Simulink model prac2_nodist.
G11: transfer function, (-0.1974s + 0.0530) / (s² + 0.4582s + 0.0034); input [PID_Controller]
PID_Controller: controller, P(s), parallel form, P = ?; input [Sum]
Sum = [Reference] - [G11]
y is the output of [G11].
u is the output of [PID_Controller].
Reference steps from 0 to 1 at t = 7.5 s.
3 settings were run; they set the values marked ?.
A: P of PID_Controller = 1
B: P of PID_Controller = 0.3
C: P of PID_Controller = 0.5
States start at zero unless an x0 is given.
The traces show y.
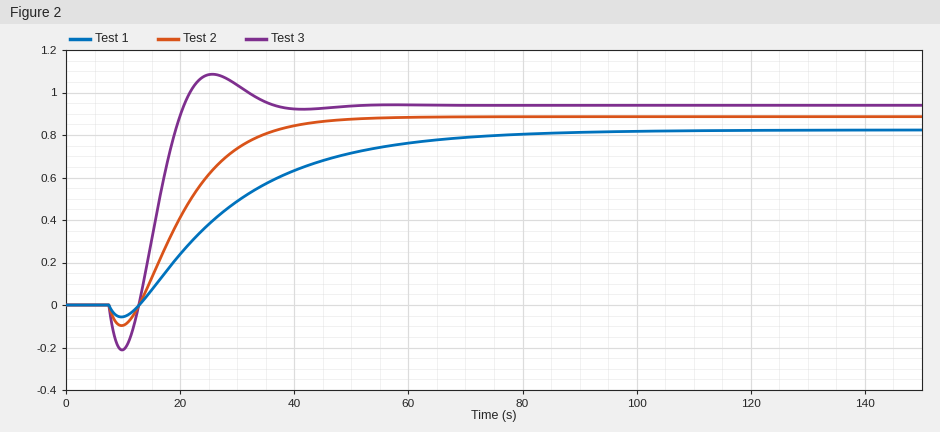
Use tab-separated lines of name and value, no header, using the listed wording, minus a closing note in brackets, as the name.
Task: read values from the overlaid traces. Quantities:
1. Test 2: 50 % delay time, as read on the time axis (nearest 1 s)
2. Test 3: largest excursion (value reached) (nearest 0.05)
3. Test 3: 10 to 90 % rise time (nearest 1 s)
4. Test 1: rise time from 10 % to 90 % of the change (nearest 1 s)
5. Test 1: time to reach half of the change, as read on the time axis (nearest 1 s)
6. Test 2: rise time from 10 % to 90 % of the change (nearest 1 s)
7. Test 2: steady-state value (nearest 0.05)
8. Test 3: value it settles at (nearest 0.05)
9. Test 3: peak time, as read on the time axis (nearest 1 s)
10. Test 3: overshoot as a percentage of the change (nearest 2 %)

Test 2: 50 % delay time, as read on the time axis	21 s
Test 3: largest excursion (value reached)	1.10
Test 3: 10 to 90 % rise time	6 s
Test 1: rise time from 10 % to 90 % of the change	40 s
Test 1: time to reach half of the change, as read on the time axis	26 s
Test 2: rise time from 10 % to 90 % of the change	20 s
Test 2: steady-state value	0.90
Test 3: value it settles at	0.95
Test 3: peak time, as read on the time axis	26 s
Test 3: overshoot as a percentage of the change	16 %
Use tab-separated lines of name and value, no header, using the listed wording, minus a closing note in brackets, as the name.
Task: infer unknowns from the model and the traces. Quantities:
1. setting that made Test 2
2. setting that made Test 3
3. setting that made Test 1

setting that made Test 2	C
setting that made Test 3	A
setting that made Test 1	B
